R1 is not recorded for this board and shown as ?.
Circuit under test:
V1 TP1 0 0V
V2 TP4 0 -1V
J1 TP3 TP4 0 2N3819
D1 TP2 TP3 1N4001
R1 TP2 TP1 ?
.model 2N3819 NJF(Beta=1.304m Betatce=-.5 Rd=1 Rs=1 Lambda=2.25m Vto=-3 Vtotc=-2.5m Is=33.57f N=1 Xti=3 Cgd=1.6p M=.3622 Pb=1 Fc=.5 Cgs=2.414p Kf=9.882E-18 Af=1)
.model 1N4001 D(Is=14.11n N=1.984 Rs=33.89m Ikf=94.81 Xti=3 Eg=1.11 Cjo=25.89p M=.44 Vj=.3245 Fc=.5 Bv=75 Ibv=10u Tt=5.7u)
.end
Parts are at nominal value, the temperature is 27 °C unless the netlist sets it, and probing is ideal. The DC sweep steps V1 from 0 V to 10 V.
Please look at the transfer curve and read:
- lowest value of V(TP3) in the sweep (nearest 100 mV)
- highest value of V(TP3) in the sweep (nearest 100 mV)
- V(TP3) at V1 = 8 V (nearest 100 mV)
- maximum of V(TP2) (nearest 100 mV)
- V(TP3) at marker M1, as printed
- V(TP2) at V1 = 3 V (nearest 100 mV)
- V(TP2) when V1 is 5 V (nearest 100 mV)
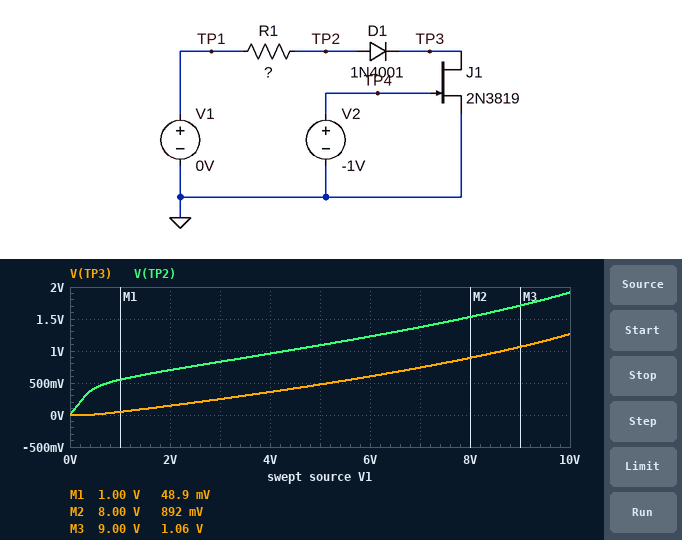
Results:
0 V
1.3 V
900 mV
1.9 V
48.9 mV
800 mV
1.1 V
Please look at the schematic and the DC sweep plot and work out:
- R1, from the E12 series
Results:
1.8 kΩ
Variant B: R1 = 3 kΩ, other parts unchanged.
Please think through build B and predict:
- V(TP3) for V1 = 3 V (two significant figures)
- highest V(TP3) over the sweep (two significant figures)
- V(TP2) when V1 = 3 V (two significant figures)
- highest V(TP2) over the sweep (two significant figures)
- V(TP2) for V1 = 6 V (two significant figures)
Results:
150 mV
670 mV
710 mV
1.3 V
960 mV
